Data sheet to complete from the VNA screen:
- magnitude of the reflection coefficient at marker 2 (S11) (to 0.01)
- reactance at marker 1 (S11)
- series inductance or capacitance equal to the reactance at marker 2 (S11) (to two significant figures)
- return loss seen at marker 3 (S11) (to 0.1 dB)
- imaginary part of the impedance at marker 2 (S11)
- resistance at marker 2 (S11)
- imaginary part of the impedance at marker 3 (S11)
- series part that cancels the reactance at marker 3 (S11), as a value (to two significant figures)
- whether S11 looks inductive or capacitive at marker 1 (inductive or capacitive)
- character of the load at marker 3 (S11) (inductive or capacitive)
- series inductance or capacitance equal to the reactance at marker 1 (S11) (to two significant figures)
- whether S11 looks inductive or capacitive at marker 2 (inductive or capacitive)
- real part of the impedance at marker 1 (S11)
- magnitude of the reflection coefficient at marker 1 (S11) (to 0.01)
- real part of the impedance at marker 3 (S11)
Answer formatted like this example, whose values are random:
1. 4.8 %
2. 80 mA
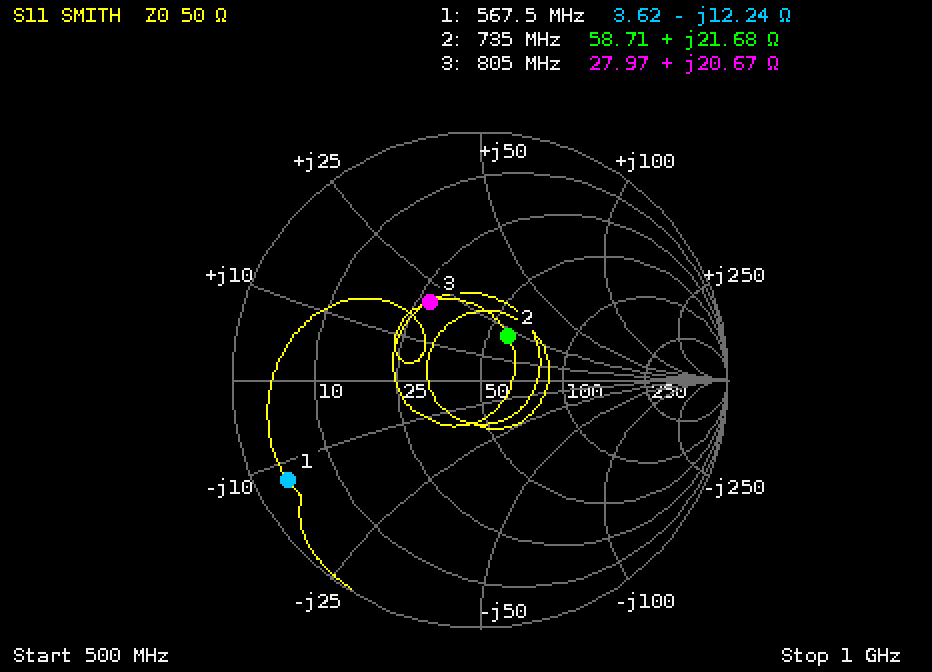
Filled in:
1. 0.21
2. -12.24 Ω
3. 4.7 nH
4. 8.5 dB
5. +21.68 Ω
6. 58.71 Ω
7. +20.67 Ω
8. 9.6 pF
9. capacitive
10. inductive
11. 23 pF
12. inductive
13. 3.62 Ω
14. 0.87
15. 27.97 Ω
